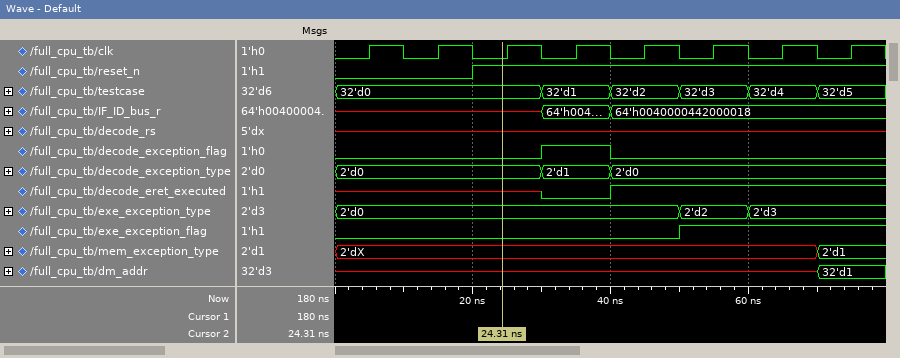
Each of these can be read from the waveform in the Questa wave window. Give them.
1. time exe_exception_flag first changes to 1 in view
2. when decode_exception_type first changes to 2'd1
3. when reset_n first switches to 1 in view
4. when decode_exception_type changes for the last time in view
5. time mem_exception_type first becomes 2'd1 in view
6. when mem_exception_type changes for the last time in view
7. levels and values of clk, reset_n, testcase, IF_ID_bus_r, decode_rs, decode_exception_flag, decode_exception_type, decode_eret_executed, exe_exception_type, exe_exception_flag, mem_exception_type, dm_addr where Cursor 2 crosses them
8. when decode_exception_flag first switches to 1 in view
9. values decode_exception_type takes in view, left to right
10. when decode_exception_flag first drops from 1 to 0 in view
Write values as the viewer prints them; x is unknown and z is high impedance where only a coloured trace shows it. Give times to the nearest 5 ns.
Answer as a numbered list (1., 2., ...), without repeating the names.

1. 50 ns
2. 30 ns
3. 20 ns
4. 40 ns
5. 70 ns
6. 70 ns
7. clk=0, reset_n=1, testcase=32'd0, IF_ID_bus_r=x, decode_rs=x, decode_exception_flag=0, decode_exception_type=2'd0, decode_eret_executed=x, exe_exception_type=2'd0, exe_exception_flag=0, mem_exception_type=2'dX, dm_addr=x
8. 30 ns
9. 2'd0, 2'd1, 2'd0
10. 40 ns
